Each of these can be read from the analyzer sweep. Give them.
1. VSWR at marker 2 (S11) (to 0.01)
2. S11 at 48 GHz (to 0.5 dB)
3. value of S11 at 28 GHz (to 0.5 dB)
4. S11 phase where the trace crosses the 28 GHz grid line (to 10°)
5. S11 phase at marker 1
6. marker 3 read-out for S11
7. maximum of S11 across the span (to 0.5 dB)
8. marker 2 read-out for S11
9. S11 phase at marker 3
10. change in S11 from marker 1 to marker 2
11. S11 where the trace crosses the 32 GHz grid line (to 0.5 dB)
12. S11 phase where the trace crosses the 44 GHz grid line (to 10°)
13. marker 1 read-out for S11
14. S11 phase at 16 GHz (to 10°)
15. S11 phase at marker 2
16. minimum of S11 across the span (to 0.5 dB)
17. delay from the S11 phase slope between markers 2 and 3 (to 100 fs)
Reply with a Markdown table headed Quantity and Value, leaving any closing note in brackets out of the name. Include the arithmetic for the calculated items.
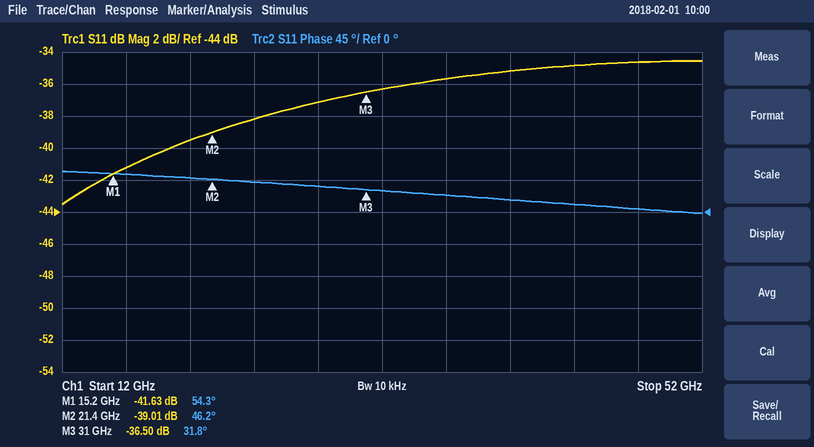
| Quantity | Value |
|---|---|
| VSWR at marker 2 (S11) | (1 + 0.0112)/(1 − 0.0112) ≈ 1.02 |
| S11 at 48 GHz | -34.5 dB |
| value of S11 at 28 GHz | -37.0 dB |
| S11 phase where the trace crosses the 28 GHz grid line | 40° |
| S11 phase at marker 1 | 54.3° |
| marker 3 read-out for S11 | -36.50 dB |
| maximum of S11 across the span | -34.5 dB |
| marker 2 read-out for S11 | -39.01 dB |
| S11 phase at marker 3 | 31.8° |
| change in S11 from marker 1 to marker 2 | -39.01 − (-41.63) = 2.62 dB |
| S11 where the trace crosses the 32 GHz grid line | -36.5 dB |
| S11 phase where the trace crosses the 44 GHz grid line | 10° |
| marker 1 read-out for S11 | -41.63 dB |
| S11 phase at 16 GHz | 50° |
| S11 phase at marker 2 | 46.2° |
| minimum of S11 across the span | -43.5 dB |
| delay from the S11 phase slope between markers 2 and 3 | −(31.8° − (46.2°))/(360° × 9.6 GHz) ≈ 4.2 ps |
